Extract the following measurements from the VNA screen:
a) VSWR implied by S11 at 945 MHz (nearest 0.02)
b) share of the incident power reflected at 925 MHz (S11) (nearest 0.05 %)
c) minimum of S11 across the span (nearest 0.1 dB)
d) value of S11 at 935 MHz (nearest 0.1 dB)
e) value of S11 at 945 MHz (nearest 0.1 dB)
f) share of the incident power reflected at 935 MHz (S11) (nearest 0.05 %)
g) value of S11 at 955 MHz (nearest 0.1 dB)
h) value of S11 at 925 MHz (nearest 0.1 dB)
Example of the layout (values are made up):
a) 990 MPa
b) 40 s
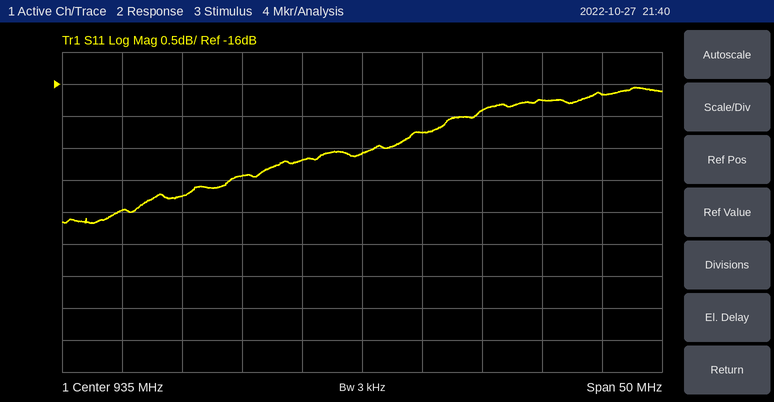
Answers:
a) 1.36
b) 1.80 %
c) -18.2 dB
d) -17.1 dB
e) -16.4 dB
f) 1.95 %
g) -16.2 dB
h) -17.4 dB
